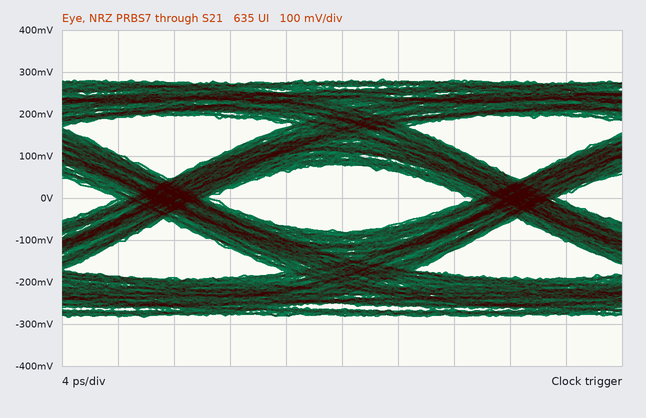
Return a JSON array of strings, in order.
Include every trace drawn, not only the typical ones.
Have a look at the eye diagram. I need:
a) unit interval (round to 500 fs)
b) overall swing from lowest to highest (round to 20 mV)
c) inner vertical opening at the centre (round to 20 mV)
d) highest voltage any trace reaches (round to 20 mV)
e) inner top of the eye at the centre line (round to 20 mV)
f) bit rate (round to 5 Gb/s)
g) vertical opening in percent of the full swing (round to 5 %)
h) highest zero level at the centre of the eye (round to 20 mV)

["25.0 ps", "560 mV", "160 mV", "280 mV", "80 mV", "40 Gb/s", "30 %", "-80 mV"]
